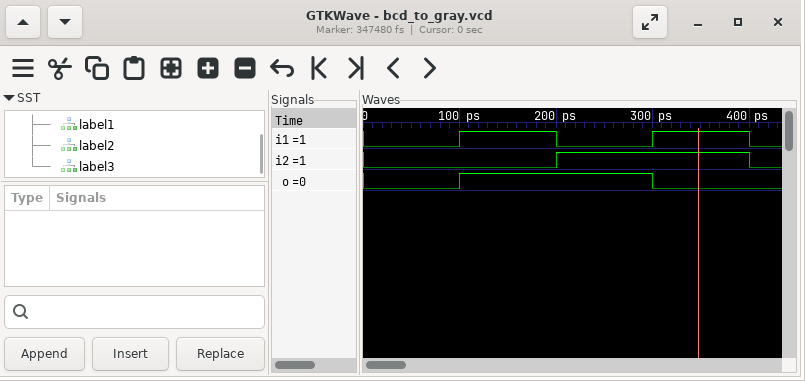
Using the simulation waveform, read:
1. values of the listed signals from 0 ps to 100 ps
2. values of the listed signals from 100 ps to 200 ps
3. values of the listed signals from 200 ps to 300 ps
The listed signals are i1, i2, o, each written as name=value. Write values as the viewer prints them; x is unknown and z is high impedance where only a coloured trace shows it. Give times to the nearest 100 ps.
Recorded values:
i1=0, i2=0, o=0
i1=1, i2=0, o=1
i1=0, i2=1, o=1
